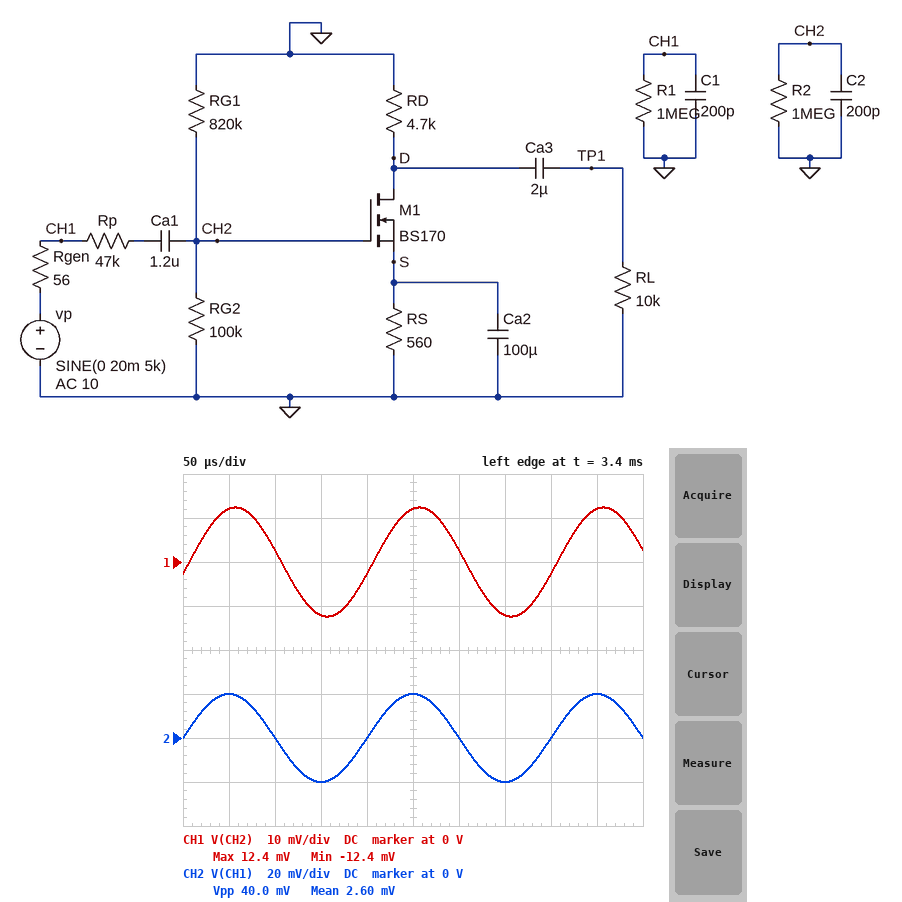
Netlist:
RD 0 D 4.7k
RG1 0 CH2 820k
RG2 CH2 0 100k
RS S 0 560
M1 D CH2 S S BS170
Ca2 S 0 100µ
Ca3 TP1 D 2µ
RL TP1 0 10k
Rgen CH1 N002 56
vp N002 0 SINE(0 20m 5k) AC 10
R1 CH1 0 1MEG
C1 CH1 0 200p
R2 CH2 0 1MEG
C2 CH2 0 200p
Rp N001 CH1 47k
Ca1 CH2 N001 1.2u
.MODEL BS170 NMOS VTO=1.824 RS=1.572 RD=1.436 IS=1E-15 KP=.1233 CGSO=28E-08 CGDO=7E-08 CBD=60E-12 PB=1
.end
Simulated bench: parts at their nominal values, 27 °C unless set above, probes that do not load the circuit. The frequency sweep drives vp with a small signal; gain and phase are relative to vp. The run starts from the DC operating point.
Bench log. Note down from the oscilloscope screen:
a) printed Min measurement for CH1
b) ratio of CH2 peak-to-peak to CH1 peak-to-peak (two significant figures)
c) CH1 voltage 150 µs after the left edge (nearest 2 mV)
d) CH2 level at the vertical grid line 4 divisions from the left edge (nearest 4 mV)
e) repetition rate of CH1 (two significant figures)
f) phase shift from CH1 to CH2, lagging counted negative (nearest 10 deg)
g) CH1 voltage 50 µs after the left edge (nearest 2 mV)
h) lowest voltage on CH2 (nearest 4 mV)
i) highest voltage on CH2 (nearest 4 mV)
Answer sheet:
-12.4 mV
1.6
-12 mV
0 V
5.0 kHz
10 deg
12 mV
-20 mV
20 mV
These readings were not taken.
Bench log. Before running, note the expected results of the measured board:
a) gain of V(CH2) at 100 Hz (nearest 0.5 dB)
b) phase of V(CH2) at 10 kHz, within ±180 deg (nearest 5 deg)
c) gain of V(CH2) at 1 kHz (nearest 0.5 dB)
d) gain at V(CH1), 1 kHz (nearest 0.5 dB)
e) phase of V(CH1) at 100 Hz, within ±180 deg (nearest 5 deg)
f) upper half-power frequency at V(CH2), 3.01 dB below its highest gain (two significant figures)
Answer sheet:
-4.0 dB
-25 deg
-4.0 dB
0 dB
0 deg
23 kHz
